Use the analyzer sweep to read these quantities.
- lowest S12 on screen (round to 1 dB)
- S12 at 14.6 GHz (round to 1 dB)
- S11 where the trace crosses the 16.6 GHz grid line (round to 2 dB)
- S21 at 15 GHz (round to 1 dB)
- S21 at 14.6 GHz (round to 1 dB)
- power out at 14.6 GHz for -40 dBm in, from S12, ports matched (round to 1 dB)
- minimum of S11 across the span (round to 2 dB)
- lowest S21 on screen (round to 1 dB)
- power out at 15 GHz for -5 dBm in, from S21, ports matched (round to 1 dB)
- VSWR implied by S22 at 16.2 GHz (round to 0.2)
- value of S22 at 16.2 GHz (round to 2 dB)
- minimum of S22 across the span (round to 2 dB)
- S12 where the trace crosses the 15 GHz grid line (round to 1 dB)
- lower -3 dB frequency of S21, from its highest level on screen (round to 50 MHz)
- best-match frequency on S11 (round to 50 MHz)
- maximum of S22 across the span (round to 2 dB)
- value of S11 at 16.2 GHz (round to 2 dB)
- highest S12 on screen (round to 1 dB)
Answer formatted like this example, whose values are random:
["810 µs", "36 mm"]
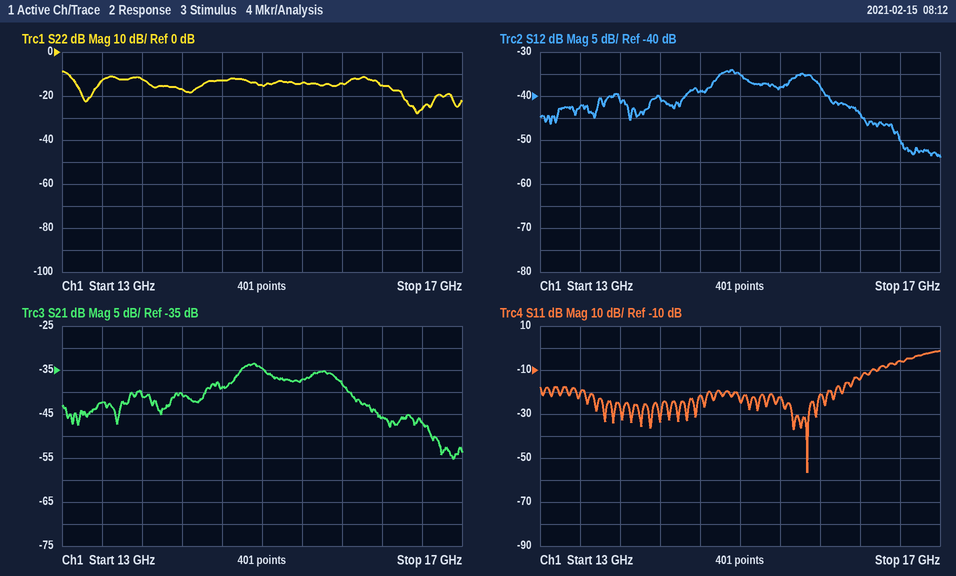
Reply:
["-54 dB", "-39 dB", "-6 dB", "-35 dB", "-39 dB", "-79 dBm", "-56 dB", "-55 dB", "-40 dBm", "1.4", "-16 dB", "-28 dB", "-35 dB", "14.75 GHz", "15.65 GHz", "-8 dB", "-14 dB", "-34 dB"]
